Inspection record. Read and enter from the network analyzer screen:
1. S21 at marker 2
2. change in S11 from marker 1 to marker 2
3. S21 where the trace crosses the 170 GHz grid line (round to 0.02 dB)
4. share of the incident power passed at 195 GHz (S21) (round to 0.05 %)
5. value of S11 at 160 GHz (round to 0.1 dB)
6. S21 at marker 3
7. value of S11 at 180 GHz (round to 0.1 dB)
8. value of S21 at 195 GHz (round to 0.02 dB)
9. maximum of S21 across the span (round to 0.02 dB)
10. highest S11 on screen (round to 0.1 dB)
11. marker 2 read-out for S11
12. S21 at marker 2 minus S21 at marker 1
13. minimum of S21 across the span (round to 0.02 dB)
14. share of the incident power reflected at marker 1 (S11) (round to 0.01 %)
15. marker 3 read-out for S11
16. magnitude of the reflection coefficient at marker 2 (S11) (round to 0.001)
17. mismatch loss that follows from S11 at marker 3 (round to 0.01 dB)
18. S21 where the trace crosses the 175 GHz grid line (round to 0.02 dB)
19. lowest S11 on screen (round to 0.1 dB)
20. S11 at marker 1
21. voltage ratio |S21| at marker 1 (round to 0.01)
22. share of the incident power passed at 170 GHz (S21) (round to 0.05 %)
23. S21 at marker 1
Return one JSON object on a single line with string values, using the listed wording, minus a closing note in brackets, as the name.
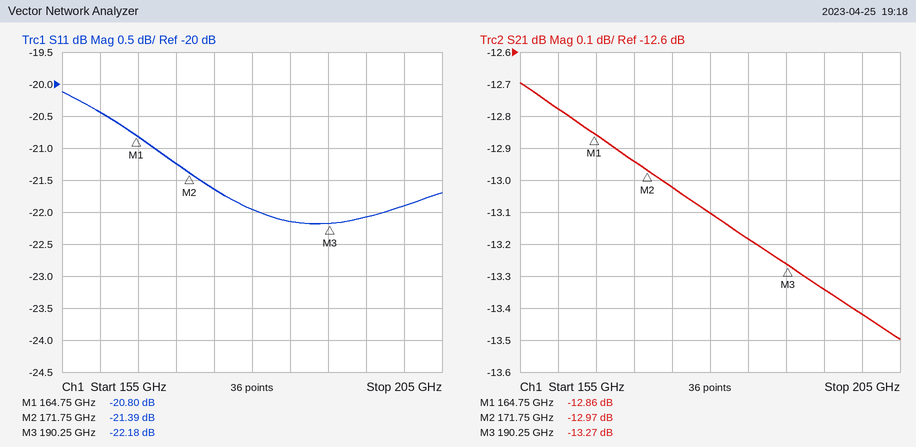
{"S21 at marker 2": "-12.97 dB", "change in S11 from marker 1 to marker 2": "-0.59 dB", "S21 where the trace crosses the 170 GHz grid line": "-12.94 dB", "share of the incident power passed at 195 GHz (S21)": "4.65 %", "value of S11 at 160 GHz": "-20.4 dB", "S21 at marker 3": "-13.27 dB", "value of S11 at 180 GHz": "-22.0 dB", "value of S21 at 195 GHz": "-13.34 dB", "maximum of S21 across the span": "-12.70 dB", "highest S11 on screen": "-20.1 dB", "marker 2 read-out for S11": "-21.39 dB", "S21 at marker 2 minus S21 at marker 1": "-0.11 dB", "minimum of S21 across the span": "-13.50 dB", "share of the incident power reflected at marker 1 (S11)": "0.83 %", "marker 3 read-out for S11": "-22.18 dB", "magnitude of the reflection coefficient at marker 2 (S11)": "0.085", "mismatch loss that follows from S11 at marker 3": "0.03 dB", "S21 where the trace crosses the 175 GHz grid line": "-13.02 dB", "lowest S11 on screen": "-22.2 dB", "S11 at marker 1": "-20.80 dB", "voltage ratio |S21| at marker 1": "0.23", "share of the incident power passed at 170 GHz (S21)": "5.10 %", "S21 at marker 1": "-12.86 dB"}
